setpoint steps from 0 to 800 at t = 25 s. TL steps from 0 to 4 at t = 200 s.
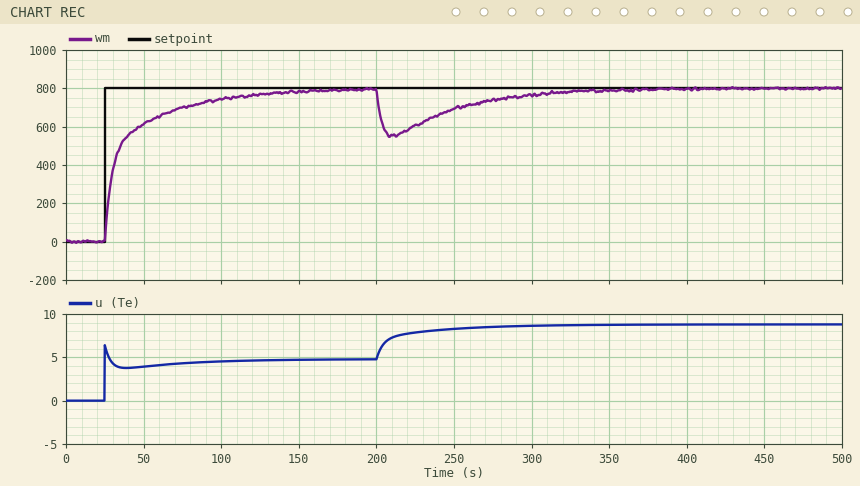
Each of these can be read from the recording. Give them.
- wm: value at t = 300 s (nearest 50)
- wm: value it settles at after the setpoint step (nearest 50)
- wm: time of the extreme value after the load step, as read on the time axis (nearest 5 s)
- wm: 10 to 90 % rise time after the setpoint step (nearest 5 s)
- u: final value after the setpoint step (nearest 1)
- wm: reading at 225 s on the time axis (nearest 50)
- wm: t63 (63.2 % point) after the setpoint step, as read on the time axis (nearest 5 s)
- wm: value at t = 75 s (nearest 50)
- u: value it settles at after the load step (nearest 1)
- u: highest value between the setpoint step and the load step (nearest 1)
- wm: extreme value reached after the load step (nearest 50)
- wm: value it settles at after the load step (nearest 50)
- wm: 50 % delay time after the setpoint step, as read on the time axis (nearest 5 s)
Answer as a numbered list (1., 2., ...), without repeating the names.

1. 750
2. 800
3. 210 s
4. 60 s
5. 5
6. 600
7. 35 s
8. 700
9. 9
10. 6
11. 550
12. 800
13. 30 s
